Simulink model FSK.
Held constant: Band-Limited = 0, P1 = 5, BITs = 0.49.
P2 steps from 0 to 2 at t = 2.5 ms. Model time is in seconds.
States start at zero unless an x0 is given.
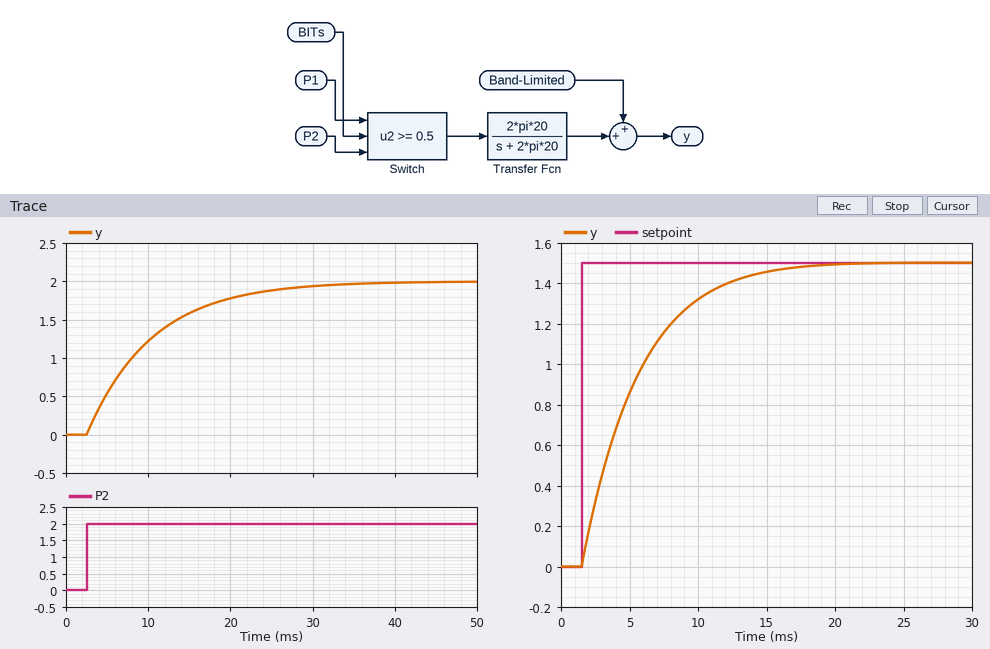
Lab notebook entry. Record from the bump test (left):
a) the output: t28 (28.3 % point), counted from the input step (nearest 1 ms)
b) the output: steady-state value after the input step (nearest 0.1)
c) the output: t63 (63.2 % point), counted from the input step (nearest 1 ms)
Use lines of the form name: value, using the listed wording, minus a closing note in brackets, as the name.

the output: t28 (28.3 % point), counted from the input step: 3 ms
the output: steady-state value after the input step: 2.0
the output: t63 (63.2 % point), counted from the input step: 8 ms
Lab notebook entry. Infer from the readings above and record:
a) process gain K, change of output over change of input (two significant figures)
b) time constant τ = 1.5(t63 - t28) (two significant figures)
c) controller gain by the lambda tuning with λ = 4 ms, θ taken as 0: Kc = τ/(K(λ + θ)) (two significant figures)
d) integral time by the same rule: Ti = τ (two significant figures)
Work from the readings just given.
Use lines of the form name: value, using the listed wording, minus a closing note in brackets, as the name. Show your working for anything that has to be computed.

process gain K, change of output over change of input: (2 - 0) / 2 = 1.0
time constant τ = 1.5(t63 - t28): 1.5 × (8 - 3) = 7.5 ms
controller gain by the lambda tuning with λ = 4 ms, θ taken as 0: Kc = τ/(K(λ + θ)): 7.5 / (1 × (4 + 0)) = 1.9
integral time by the same rule: Ti = τ: 7.5 ms
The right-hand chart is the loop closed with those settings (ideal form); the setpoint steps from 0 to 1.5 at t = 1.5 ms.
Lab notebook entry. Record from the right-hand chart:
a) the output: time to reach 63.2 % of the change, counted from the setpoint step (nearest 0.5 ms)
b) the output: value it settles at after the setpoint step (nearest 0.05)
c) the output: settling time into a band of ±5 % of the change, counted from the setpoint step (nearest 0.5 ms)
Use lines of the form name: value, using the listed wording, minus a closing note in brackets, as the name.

the output: time to reach 63.2 % of the change, counted from the setpoint step: 4.0 ms
the output: value it settles at after the setpoint step: 1.50
the output: settling time into a band of ±5 % of the change, counted from the setpoint step: 11.5 ms
